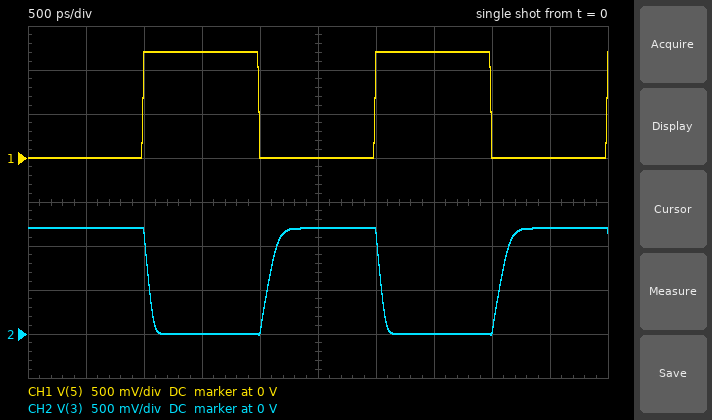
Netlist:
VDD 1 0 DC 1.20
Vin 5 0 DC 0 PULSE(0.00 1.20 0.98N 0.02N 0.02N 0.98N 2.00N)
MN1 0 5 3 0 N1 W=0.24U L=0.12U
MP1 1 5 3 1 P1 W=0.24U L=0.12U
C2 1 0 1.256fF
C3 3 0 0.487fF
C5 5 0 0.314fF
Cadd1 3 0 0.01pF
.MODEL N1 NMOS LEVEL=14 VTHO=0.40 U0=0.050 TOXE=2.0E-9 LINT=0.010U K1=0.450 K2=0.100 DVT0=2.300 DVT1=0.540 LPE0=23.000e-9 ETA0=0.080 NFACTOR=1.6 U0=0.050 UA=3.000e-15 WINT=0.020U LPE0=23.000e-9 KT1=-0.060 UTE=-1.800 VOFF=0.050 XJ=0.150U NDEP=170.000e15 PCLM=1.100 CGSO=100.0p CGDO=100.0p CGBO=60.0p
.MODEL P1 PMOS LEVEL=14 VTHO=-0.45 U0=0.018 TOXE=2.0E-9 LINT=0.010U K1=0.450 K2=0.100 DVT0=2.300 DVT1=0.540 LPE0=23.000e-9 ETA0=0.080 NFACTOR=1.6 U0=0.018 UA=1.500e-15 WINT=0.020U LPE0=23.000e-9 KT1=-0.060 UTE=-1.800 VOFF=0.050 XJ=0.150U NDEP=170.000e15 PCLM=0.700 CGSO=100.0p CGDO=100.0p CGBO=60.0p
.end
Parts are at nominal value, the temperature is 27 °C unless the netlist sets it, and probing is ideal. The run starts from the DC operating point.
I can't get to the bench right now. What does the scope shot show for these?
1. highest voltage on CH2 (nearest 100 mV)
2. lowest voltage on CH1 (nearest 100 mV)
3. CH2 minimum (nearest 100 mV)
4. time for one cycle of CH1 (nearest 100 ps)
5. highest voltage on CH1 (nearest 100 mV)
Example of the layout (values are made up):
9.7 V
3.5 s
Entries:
1.2 V
0 V
0 V
2.0 ns
1.2 V
